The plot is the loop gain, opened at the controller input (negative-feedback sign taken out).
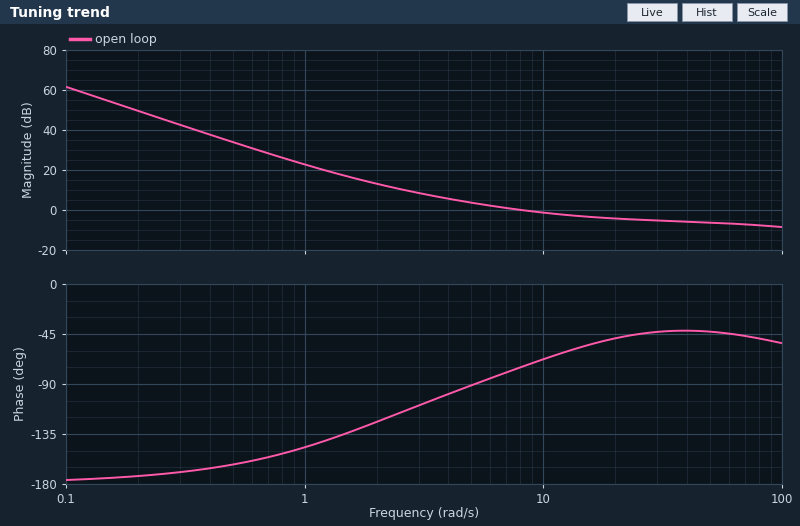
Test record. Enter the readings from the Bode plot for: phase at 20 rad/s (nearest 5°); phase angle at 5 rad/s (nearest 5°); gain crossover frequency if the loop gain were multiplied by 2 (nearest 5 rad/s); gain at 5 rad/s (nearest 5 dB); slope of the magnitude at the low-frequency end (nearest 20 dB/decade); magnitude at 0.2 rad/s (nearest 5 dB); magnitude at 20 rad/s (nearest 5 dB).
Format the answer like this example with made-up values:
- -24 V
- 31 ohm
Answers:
- -50°
- -90°
- 45 rad/s
- 5 dB
- -40 dB/decade
- 50 dB
- -5 dB
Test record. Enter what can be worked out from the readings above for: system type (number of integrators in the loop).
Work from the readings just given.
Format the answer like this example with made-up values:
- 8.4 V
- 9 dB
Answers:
- 2
